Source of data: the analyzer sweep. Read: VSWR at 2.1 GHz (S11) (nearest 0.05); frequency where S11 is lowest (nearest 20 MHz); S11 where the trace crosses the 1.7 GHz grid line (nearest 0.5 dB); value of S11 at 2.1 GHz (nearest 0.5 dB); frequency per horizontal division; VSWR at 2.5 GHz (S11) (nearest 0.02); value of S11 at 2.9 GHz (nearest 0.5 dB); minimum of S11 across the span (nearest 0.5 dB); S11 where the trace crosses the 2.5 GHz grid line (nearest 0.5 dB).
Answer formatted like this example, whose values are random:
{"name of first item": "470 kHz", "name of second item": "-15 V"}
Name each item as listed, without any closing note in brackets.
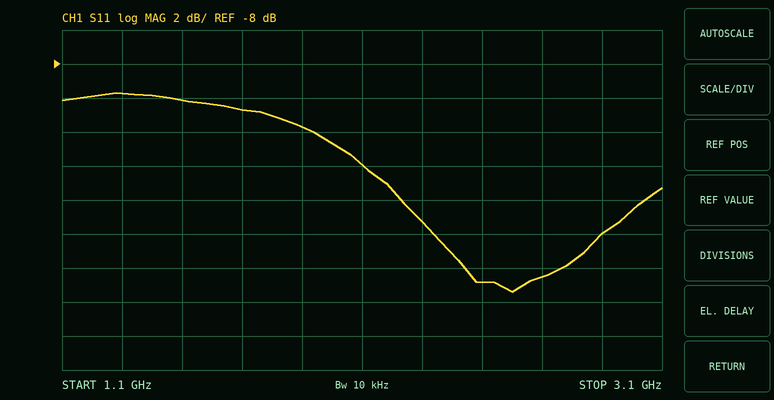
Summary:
{"VSWR at 2.1 GHz (S11)": "1.50", "frequency where S11 is lowest": "2.60 GHz", "S11 where the trace crosses the 1.7 GHz grid line": "-10.5 dB", "value of S11 at 2.1 GHz": "-14.0 dB", "frequency per horizontal division": "200 MHz", "VSWR at 2.5 GHz (S11)": "1.20", "value of S11 at 2.9 GHz": "-18.0 dB", "minimum of S11 across the span": "-21.5 dB", "S11 where the trace crosses the 2.5 GHz grid line": "-21.0 dB"}
